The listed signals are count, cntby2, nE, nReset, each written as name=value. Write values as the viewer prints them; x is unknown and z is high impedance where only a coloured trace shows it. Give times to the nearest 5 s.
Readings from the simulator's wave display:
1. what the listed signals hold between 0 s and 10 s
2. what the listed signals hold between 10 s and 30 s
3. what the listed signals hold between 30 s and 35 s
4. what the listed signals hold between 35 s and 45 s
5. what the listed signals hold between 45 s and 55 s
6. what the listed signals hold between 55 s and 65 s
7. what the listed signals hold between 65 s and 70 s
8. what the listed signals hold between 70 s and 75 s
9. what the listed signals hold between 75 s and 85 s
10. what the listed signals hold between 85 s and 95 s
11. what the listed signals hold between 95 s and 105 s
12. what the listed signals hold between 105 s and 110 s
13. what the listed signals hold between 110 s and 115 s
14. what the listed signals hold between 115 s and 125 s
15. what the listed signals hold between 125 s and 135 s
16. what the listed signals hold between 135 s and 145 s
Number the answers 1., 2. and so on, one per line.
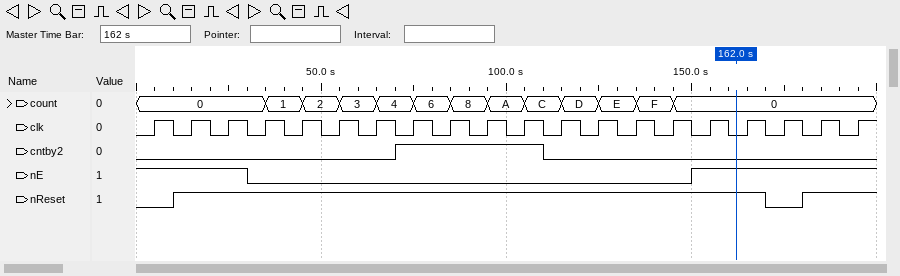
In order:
1. count=0, cntby2=0, nE=1, nReset=0
2. count=0, cntby2=0, nE=1, nReset=1
3. count=0, cntby2=0, nE=0, nReset=1
4. count=1, cntby2=0, nE=0, nReset=1
5. count=2, cntby2=0, nE=0, nReset=1
6. count=3, cntby2=0, nE=0, nReset=1
7. count=4, cntby2=0, nE=0, nReset=1
8. count=4, cntby2=1, nE=0, nReset=1
9. count=6, cntby2=1, nE=0, nReset=1
10. count=8, cntby2=1, nE=0, nReset=1
11. count=A, cntby2=1, nE=0, nReset=1
12. count=C, cntby2=1, nE=0, nReset=1
13. count=C, cntby2=0, nE=0, nReset=1
14. count=D, cntby2=0, nE=0, nReset=1
15. count=E, cntby2=0, nE=0, nReset=1
16. count=F, cntby2=0, nE=0, nReset=1
